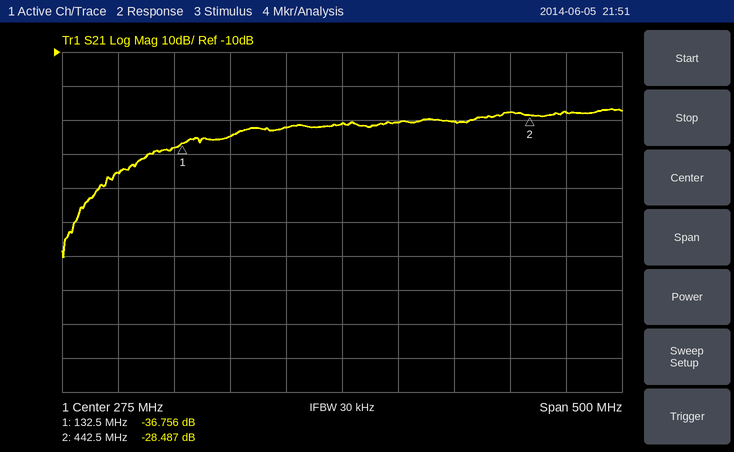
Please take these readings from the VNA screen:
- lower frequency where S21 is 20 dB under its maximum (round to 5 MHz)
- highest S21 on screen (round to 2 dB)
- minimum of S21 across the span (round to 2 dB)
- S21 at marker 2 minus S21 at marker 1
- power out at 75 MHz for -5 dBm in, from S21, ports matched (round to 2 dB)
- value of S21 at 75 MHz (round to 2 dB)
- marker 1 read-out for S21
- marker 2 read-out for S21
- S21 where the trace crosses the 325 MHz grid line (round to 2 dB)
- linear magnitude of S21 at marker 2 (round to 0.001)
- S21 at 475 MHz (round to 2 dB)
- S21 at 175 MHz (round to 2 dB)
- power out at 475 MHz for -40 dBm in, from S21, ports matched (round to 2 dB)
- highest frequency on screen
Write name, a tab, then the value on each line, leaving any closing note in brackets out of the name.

lower frequency where S21 is 20 dB under its maximum	70 MHz
highest S21 on screen	-26 dB
minimum of S21 across the span	-70 dB
S21 at marker 2 minus S21 at marker 1	8.269 dB
power out at 75 MHz for -5 dBm in, from S21, ports matched	-50 dBm
value of S21 at 75 MHz	-46 dB
marker 1 read-out for S21	-36.756 dB
marker 2 read-out for S21	-28.487 dB
S21 where the trace crosses the 325 MHz grid line	-30 dB
linear magnitude of S21 at marker 2	0.038
S21 at 475 MHz	-28 dB
S21 at 175 MHz	-34 dB
power out at 475 MHz for -40 dBm in, from S21, ports matched	-68 dBm
highest frequency on screen	525 MHz
